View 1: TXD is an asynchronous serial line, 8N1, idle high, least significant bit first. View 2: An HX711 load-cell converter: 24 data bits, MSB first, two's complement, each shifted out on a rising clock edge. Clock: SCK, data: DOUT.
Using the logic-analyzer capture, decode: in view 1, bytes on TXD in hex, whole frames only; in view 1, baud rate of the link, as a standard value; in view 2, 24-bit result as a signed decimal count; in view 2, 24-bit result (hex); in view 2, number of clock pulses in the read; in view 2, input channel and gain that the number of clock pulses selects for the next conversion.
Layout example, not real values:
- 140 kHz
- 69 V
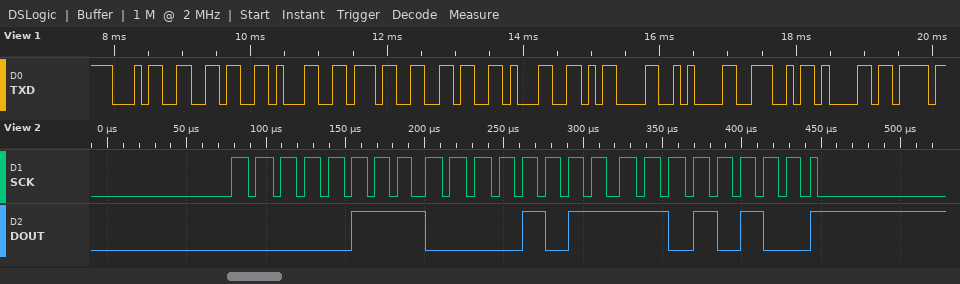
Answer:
- 34 36 31 37 36 31 0D 0A 4E 61
- 9600 baud
- 461780
- 0x070BD4
- 25
- channel A, gain 128
